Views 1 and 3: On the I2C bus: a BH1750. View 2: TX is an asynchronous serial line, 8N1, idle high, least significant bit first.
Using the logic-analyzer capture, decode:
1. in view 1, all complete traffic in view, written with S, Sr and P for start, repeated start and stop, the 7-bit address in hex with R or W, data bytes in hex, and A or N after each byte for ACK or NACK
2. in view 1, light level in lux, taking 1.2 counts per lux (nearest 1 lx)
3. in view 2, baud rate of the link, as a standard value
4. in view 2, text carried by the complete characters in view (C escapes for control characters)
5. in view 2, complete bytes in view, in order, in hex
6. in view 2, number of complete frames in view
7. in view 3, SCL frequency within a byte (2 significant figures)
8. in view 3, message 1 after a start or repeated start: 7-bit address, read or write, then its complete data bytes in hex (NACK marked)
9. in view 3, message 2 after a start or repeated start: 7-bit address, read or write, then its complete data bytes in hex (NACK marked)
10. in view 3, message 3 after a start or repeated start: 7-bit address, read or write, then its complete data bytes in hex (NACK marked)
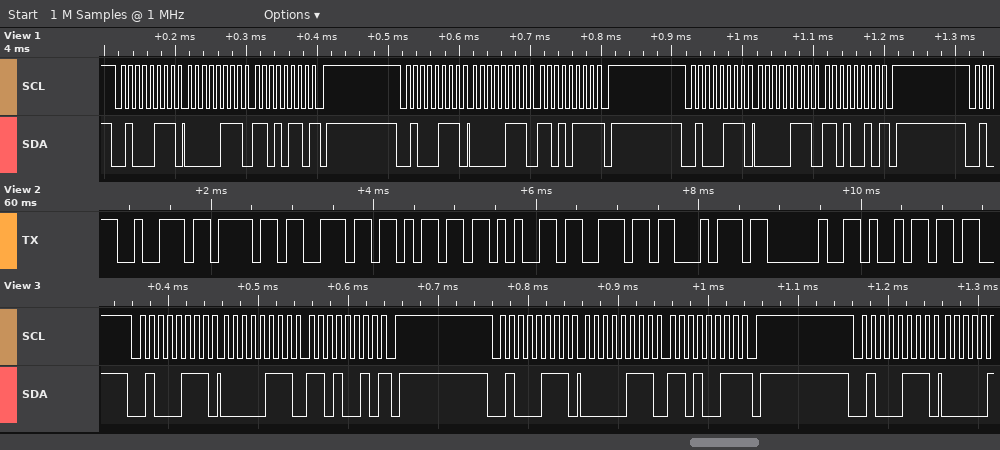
S 23R A 07 A D6 N P S 23R A 07 A D7 N P S 23R A 07 A D2 N P
1672 lx
9600 baud
"ronment i"
72 6F 6E 6D 65 6E 74 20 69
9
100 kHz
0x23 read: 07 D2 NACK
0x23 read: 07 D3 NACK
0x23 read
